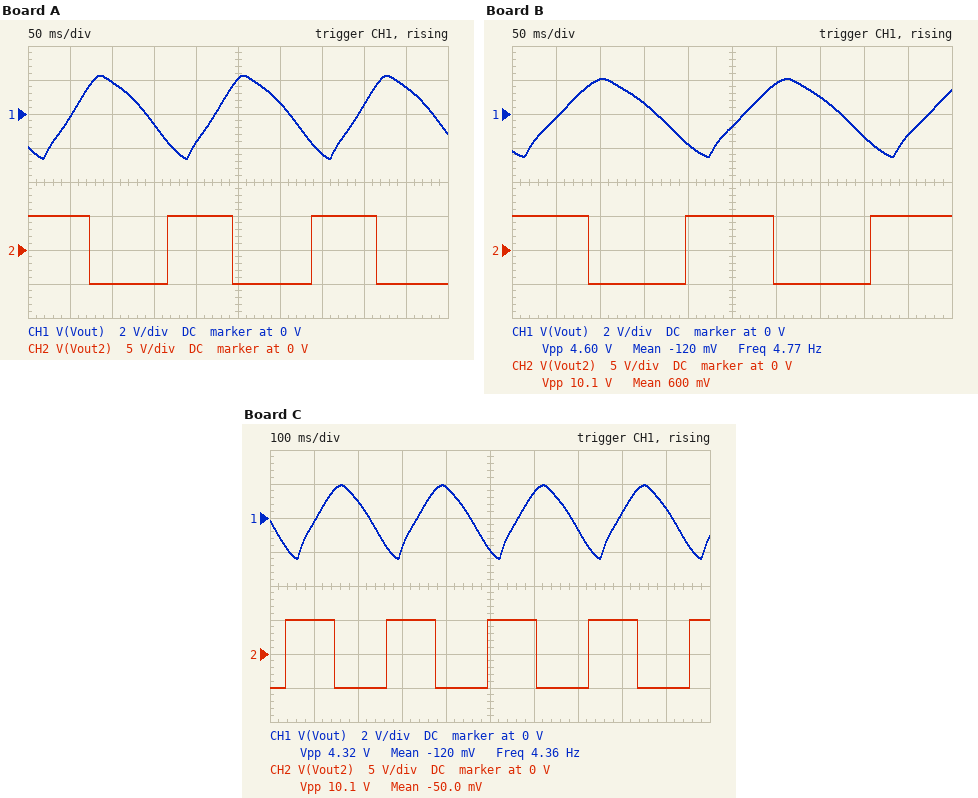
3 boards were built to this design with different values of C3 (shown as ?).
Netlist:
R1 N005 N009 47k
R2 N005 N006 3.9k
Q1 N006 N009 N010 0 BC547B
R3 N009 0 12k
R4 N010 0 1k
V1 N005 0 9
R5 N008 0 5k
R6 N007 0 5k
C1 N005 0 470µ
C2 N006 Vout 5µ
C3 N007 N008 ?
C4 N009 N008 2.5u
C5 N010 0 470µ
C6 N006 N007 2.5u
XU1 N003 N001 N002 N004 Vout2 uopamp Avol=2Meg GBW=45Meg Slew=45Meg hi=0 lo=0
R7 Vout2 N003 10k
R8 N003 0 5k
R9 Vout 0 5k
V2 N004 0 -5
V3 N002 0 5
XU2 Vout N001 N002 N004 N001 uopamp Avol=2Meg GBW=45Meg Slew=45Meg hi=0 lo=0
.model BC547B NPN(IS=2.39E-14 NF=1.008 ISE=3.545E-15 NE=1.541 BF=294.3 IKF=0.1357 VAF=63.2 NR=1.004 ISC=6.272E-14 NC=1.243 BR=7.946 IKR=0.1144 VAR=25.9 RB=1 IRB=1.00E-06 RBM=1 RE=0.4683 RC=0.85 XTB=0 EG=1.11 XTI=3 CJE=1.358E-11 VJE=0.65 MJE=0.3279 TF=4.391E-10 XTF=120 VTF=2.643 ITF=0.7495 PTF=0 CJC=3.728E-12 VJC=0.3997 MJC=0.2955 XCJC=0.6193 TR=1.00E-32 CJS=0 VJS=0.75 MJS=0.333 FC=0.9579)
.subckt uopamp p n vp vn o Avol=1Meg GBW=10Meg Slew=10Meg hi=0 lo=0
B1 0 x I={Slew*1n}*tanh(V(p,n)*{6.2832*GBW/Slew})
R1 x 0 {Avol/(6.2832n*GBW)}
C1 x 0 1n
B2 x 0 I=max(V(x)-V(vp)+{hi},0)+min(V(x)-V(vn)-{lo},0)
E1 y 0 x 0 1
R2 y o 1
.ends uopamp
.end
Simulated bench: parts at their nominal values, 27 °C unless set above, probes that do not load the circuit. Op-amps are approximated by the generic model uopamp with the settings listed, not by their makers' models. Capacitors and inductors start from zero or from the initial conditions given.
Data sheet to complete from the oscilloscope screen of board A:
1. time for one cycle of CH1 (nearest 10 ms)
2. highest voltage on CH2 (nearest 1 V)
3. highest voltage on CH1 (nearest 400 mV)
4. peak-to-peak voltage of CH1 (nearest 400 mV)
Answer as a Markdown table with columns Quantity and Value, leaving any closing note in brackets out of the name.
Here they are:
| Quantity | Value |
|---|---|
| time for one cycle of CH1 | 170 ms |
| highest voltage on CH2 | 5 V |
| highest voltage on CH1 | 2.4 V |
| peak-to-peak voltage of CH1 | 4.8 V |
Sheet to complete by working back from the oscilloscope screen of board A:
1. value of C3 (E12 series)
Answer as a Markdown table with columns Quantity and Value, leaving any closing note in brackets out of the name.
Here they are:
| Quantity | Value |
|---|---|
| value of C3 | 1.8 µF |
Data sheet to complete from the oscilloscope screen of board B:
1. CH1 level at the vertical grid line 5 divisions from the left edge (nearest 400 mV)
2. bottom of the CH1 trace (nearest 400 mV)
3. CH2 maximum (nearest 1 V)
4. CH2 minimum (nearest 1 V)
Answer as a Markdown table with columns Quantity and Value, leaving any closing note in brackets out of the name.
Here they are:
| Quantity | Value |
|---|---|
| CH1 level at the vertical grid line 5 divisions from the left edge | -800 mV |
| bottom of the CH1 trace | -2.4 V |
| CH2 maximum | 5 V |
| CH2 minimum | -5 V |
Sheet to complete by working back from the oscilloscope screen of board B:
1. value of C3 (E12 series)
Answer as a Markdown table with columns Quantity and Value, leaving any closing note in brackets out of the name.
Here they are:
| Quantity | Value |
|---|---|
| value of C3 | 3.9 µF |
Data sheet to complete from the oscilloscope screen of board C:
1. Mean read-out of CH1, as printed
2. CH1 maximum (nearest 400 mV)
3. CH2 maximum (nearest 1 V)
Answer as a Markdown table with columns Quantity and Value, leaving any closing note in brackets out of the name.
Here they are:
| Quantity | Value |
|---|---|
| Mean read-out of CH1, as printed | -120 mV |
| CH1 maximum | 2.0 V |
| CH2 maximum | 5 V |
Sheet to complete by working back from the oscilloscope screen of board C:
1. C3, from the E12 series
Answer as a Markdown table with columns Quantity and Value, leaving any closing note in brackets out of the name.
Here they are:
| Quantity | Value |
|---|---|
| C3, from the E12 series | 5.6 µF |
